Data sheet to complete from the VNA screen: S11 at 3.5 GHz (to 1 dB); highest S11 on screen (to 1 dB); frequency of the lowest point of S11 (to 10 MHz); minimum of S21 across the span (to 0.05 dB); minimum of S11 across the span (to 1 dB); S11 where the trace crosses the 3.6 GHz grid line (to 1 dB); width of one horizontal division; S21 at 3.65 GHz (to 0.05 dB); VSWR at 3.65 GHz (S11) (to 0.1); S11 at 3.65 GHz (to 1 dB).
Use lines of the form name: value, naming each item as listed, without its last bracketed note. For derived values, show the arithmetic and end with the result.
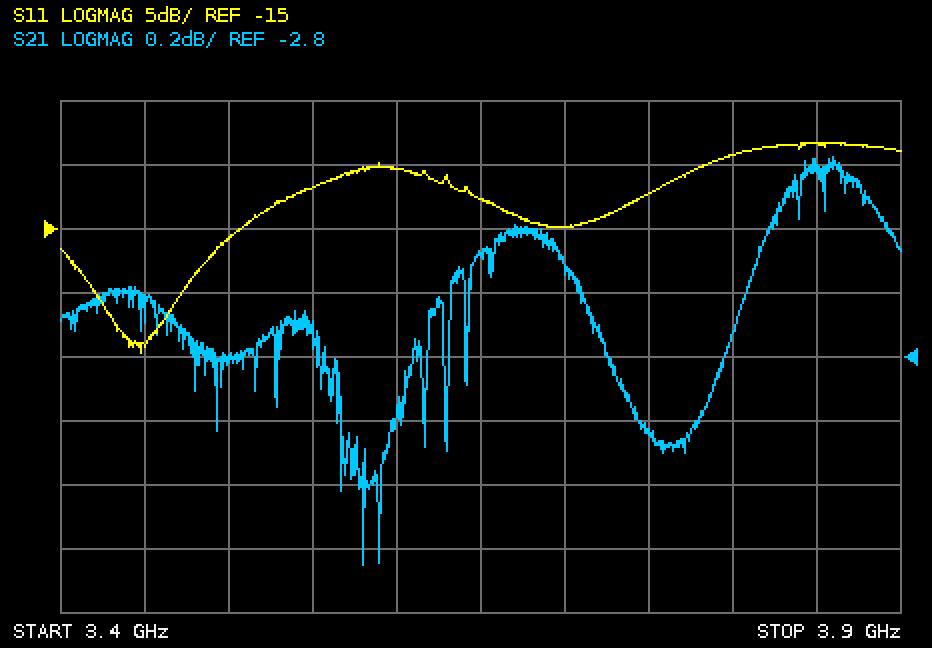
S11 at 3.5 GHz: -16 dB
highest S11 on screen: -8 dB
frequency of the lowest point of S11: 3.45 GHz
minimum of S21 across the span: -3.45 dB
minimum of S11 across the span: -25 dB
S11 where the trace crosses the 3.6 GHz grid line: -10 dB
width of one horizontal division: 50 MHz
S21 at 3.65 GHz: -2.50 dB
VSWR at 3.65 GHz (S11): |Γ| = 10^(-13/20) = 0.2239; VSWR = (1 + 0.2239)/(1 − 0.2239) ≈ 1.6
S11 at 3.65 GHz: -13 dB
